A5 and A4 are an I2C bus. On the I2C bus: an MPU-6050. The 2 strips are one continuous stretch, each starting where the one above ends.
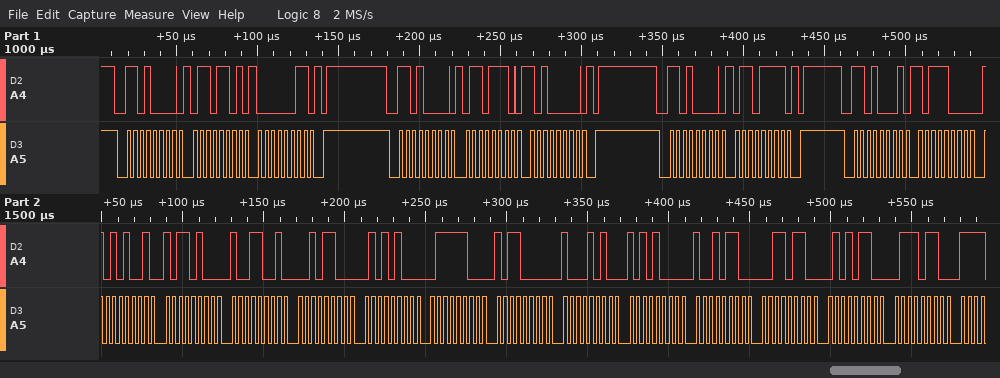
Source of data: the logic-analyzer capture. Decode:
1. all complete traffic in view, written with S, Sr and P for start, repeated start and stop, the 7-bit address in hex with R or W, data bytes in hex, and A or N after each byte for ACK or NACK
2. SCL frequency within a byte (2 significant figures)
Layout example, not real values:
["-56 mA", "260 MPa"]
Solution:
["S 68W A 6D A 03 A P S 68W A 6E A A0 A P S 68W A 6F A P S 68R A B8 A A9 A B4 A 99 A 2C A 54 A 7C A B0 A 8A A A8 A 96 A 36 A 56 A 76 A", "250 kHz"]
